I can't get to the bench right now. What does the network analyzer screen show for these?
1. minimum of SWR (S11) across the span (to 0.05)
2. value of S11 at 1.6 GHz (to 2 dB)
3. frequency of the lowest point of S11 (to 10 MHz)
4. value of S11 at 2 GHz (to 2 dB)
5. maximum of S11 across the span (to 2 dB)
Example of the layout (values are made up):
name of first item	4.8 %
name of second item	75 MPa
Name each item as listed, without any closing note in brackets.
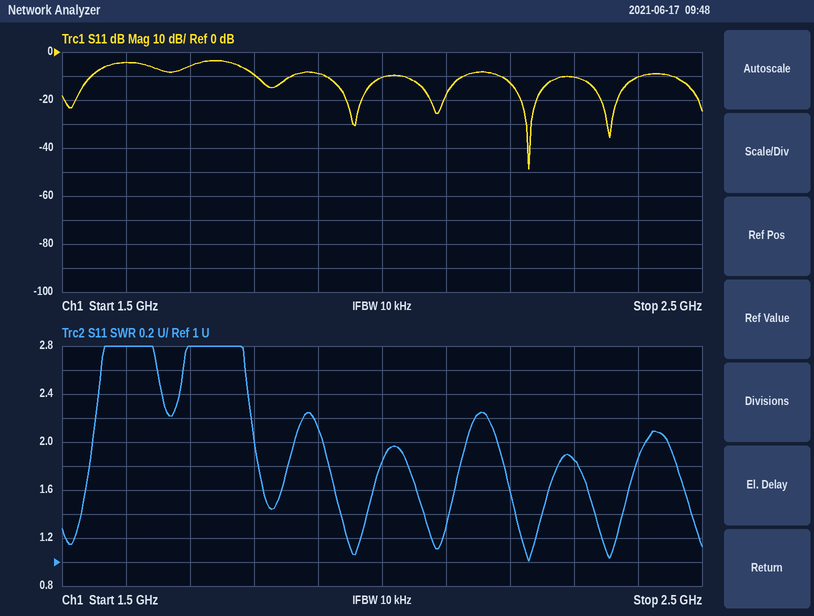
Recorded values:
minimum of SWR (S11) across the span	1.00
value of S11 at 1.6 GHz	-4 dB
frequency of the lowest point of S11	2.23 GHz
value of S11 at 2 GHz	-10 dB
maximum of S11 across the span	-4 dB
